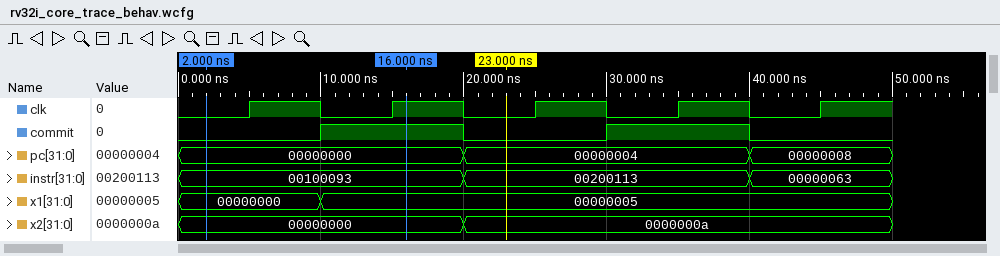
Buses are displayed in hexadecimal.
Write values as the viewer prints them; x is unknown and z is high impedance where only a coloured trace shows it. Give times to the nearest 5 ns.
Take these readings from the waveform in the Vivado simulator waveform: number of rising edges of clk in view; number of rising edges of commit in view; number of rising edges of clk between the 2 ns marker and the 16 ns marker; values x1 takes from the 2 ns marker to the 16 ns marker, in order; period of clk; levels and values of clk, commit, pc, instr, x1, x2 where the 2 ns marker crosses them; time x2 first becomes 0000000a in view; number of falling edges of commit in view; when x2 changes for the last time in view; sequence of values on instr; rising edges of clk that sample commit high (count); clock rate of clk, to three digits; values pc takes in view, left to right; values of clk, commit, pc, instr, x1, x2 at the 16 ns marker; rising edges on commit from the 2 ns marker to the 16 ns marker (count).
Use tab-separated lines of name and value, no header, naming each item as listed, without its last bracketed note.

number of rising edges of clk in view	5
number of rising edges of commit in view	2
number of rising edges of clk between the 2 ns marker and the 16 ns marker	2
values x1 takes from the 2 ns marker to the 16 ns marker, in order	00000000, 00000005
period of clk	10 ns
levels and values of clk, commit, pc, instr, x1, x2 where the 2 ns marker crosses them	clk=0, commit=0, pc=00000000, instr=00100093, x1=00000000, x2=00000000
time x2 first becomes 0000000a in view	20 ns
number of falling edges of commit in view	2
when x2 changes for the last time in view	20 ns
sequence of values on instr	00100093, 00200113, 00000063
rising edges of clk that sample commit high	2
clock rate of clk, to three digits	100 MHz
values pc takes in view, left to right	00000000, 00000004, 00000008
values of clk, commit, pc, instr, x1, x2 at the 16 ns marker	clk=1, commit=1, pc=00000000, instr=00100093, x1=00000005, x2=00000000
rising edges on commit from the 2 ns marker to the 16 ns marker	1
